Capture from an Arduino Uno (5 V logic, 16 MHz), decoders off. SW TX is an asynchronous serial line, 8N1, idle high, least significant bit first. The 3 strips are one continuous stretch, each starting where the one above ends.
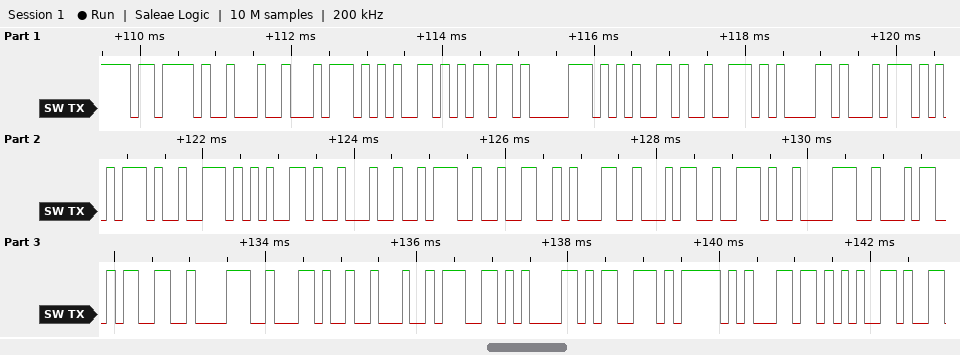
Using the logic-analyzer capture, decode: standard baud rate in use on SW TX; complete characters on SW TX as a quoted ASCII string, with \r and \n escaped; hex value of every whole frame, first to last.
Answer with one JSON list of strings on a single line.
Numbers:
["9600 baud", "\"{\\\"temperature\\\":214.8438,\\\"gas_le\"", "0x7B 0x22 0x74 0x65 0x6D 0x70 0x65 0x72 0x61 0x74 0x75 0x72 0x65 0x22 0x3A 0x32 0x31 0x34 0x2E 0x38 0x34 0x33 0x38 0x2C 0x22 0x67 0x61 0x73 0x5F 0x6C 0x65"]
